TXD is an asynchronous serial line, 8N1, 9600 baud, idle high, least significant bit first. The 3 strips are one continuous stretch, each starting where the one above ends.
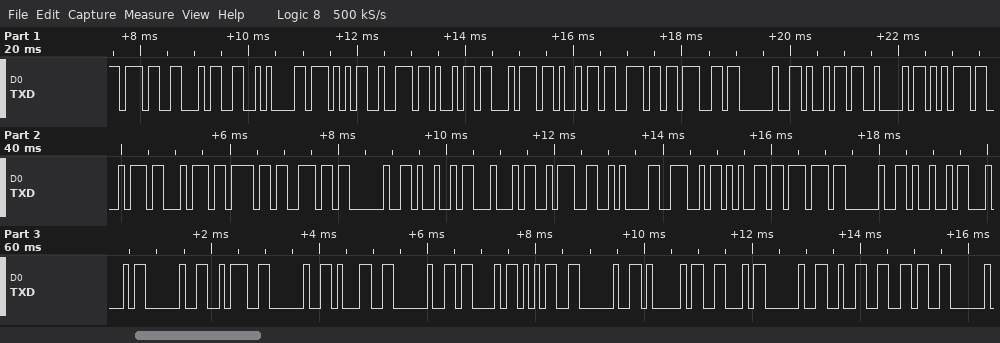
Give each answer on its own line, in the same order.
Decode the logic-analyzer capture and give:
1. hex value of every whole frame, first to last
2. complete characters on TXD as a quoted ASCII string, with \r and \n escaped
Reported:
37 34 0A 57 72 69 74 69 6E 67 20 69 42 75 74 74 6F 6E 20 49 44 3A 0A 4E 65 77 20 49 44 20 3A 20 31 20 43 35 20 41 46 20 32 36
"74\nWriting iButton ID:\nNew ID : 1 C5 AF 26"
